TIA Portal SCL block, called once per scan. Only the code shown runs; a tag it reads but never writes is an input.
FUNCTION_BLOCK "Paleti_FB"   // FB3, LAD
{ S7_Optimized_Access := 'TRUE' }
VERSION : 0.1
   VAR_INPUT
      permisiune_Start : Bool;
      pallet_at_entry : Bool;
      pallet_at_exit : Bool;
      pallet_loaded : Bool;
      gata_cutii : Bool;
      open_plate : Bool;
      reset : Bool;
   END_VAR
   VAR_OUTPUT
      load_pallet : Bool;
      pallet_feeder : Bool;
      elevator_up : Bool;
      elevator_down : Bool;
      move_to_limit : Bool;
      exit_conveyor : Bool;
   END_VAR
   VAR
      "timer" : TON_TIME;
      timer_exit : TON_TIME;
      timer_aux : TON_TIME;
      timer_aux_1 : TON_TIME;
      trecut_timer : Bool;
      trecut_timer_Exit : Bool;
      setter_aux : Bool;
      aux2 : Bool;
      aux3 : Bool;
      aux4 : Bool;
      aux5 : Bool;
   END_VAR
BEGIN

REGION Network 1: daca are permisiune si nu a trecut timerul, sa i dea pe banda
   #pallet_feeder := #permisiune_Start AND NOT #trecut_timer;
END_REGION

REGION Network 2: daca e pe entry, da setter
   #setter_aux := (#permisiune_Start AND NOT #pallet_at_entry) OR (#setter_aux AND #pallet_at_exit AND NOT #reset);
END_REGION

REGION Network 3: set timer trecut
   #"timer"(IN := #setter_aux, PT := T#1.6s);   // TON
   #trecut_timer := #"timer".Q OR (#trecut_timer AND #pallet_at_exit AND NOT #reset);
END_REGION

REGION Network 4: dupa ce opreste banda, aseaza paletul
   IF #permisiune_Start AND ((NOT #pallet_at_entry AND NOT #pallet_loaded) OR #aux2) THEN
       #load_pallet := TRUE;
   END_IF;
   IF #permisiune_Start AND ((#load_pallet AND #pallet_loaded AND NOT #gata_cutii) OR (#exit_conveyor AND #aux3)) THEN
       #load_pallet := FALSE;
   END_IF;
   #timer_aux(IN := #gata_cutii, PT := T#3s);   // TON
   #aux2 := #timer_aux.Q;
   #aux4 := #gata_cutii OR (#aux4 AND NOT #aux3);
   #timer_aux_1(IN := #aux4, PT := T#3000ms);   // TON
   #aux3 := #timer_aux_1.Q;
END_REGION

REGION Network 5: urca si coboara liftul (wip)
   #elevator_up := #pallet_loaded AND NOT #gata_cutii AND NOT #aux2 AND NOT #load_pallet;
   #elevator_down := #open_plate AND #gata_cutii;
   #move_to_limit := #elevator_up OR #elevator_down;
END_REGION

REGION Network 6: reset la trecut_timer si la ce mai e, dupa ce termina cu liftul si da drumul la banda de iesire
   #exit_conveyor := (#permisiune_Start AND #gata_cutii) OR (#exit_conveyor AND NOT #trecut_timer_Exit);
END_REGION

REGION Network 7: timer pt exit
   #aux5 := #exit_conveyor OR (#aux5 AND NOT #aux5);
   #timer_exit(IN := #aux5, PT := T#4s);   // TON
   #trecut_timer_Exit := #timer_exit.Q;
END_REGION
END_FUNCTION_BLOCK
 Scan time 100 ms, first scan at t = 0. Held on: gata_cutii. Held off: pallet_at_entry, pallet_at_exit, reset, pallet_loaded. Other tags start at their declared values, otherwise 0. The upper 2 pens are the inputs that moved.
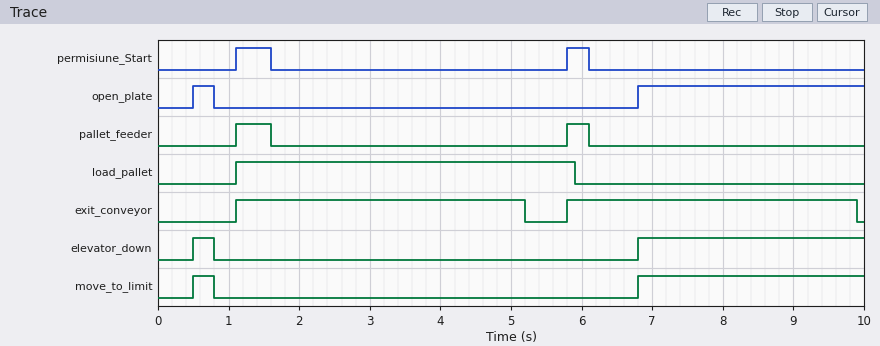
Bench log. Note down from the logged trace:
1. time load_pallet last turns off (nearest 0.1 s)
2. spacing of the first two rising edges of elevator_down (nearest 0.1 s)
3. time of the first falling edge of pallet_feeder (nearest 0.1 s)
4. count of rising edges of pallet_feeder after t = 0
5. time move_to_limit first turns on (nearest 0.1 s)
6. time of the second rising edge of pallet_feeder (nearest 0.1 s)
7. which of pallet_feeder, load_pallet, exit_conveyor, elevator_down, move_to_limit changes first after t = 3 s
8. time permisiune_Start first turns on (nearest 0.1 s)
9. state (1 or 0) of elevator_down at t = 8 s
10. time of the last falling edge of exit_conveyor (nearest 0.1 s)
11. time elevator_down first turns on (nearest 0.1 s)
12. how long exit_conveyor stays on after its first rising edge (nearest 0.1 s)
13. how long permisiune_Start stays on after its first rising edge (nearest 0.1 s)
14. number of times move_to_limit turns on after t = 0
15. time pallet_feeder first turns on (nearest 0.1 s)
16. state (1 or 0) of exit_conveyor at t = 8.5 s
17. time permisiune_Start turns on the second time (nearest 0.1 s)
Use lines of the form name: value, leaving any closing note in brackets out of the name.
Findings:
time load_pallet last turns off: 5.9 s
spacing of the first two rising edges of elevator_down: 6.3 s
time of the first falling edge of pallet_feeder: 1.6 s
count of rising edges of pallet_feeder after t = 0: 2
time move_to_limit first turns on: 0.5 s
time of the second rising edge of pallet_feeder: 5.8 s
which of pallet_feeder, load_pallet, exit_conveyor, elevator_down, move_to_limit changes first after t = 3 s: exit_conveyor
time permisiune_Start first turns on: 1.1 s
state (1 or 0) of elevator_down at t = 8 s: 1
time of the last falling edge of exit_conveyor: 9.9 s
time elevator_down first turns on: 0.5 s
how long exit_conveyor stays on after its first rising edge: 4.1 s
how long permisiune_Start stays on after its first rising edge: 0.5 s
number of times move_to_limit turns on after t = 0: 2
time pallet_feeder first turns on: 1.1 s
state (1 or 0) of exit_conveyor at t = 8.5 s: 1
time permisiune_Start turns on the second time: 5.8 s
